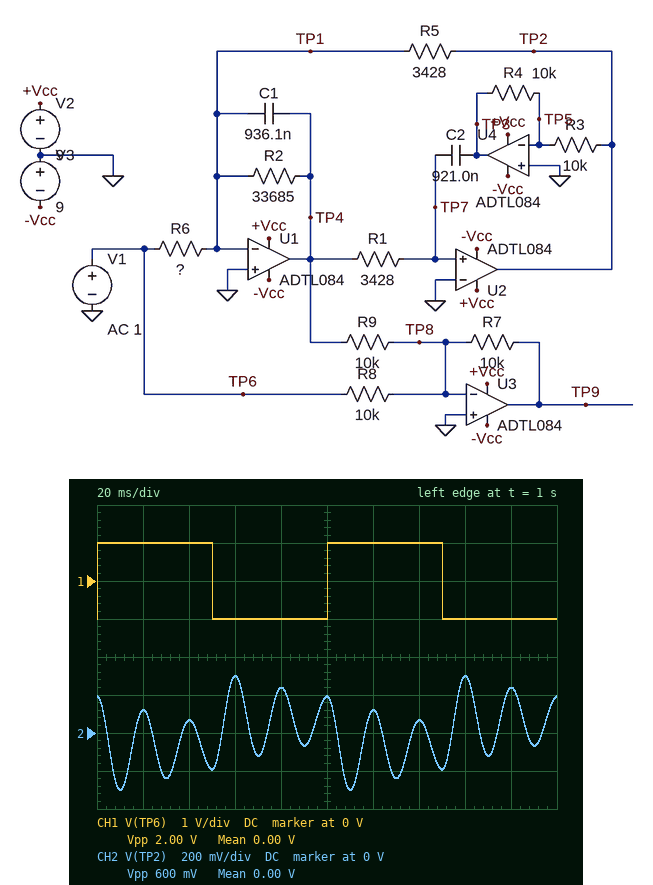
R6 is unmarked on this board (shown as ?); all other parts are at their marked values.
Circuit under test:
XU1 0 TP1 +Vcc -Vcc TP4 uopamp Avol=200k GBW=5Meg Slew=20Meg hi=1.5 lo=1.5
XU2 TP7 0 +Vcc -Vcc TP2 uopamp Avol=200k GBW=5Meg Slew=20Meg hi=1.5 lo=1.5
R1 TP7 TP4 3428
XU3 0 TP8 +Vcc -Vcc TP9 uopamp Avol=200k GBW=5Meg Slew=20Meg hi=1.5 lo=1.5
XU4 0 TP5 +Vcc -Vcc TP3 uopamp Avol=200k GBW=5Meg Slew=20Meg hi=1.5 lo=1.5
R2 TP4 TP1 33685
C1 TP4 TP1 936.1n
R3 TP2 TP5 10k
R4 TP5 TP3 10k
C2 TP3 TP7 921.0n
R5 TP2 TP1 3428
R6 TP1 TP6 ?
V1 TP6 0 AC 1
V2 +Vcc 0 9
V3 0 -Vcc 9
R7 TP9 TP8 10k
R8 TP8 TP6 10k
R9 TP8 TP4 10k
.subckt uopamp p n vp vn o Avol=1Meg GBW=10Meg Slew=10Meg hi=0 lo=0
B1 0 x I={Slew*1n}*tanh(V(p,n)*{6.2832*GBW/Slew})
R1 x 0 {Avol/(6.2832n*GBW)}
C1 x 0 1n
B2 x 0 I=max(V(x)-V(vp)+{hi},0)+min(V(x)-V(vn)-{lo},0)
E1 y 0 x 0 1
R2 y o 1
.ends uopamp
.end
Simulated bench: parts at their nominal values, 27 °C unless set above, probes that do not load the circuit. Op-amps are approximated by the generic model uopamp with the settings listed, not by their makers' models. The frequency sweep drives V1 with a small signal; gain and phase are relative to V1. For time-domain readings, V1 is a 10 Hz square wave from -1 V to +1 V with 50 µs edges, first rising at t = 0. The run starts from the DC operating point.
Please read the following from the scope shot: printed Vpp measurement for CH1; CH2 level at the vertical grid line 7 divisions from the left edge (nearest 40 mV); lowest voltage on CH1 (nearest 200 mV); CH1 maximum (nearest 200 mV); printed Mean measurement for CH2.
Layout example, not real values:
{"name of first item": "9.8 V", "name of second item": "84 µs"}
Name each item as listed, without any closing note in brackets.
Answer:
{"printed Vpp measurement for CH1": "2.00 V", "CH2 level at the vertical grid line 7 divisions from the left edge": "80 mV", "lowest voltage on CH1": "-1.0 V", "CH1 maximum": "1.0 V", "printed Mean measurement for CH2": "0.00 V"}
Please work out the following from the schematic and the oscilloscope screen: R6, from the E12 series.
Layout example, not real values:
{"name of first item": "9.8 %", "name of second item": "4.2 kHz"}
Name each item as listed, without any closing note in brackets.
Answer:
{"R6, from the E12 series": "47 kΩ"}
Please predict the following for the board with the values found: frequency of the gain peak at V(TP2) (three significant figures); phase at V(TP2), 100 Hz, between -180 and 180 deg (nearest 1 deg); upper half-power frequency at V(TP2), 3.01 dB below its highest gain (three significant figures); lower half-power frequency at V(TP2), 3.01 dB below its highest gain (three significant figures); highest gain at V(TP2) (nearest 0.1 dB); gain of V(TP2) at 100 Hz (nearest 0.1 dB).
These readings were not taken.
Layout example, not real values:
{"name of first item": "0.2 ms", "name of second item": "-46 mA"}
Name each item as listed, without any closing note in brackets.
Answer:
{"frequency of the gain peak at V(TP2)": "49.9 Hz", "phase at V(TP2), 100 Hz, between -180 and 180 deg": "4 deg", "upper half-power frequency at V(TP2), 3.01 dB below its highest gain": "52.3 Hz", "lower half-power frequency at V(TP2), 3.01 dB below its highest gain": "47.3 Hz", "highest gain at V(TP2)": "-2.8 dB", "gain of V(TP2) at 100 Hz": "-32.3 dB"}
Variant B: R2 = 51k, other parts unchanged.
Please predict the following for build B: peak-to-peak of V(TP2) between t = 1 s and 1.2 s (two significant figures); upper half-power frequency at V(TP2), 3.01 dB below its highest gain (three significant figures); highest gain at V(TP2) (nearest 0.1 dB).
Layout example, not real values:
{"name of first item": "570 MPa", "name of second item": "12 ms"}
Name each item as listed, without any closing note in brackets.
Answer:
{"peak-to-peak of V(TP2) between t = 1 s and 1.2 s": "790 mV", "upper half-power frequency at V(TP2), 3.01 dB below its highest gain": "51.6 Hz", "highest gain at V(TP2)": "0.8 dB"}
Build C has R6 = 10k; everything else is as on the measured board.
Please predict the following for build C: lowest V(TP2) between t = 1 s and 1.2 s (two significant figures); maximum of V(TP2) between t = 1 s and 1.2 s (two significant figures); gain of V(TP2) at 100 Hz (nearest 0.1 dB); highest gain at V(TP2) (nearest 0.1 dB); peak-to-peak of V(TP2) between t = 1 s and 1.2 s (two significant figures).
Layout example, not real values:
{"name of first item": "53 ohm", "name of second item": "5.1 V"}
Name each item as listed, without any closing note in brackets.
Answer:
{"lowest V(TP2) between t = 1 s and 1.2 s": "-1.4 V", "maximum of V(TP2) between t = 1 s and 1.2 s": "1.4 V", "gain of V(TP2) at 100 Hz": "-18.9 dB", "highest gain at V(TP2)": "10.6 dB", "peak-to-peak of V(TP2) between t = 1 s and 1.2 s": "2.8 V"}
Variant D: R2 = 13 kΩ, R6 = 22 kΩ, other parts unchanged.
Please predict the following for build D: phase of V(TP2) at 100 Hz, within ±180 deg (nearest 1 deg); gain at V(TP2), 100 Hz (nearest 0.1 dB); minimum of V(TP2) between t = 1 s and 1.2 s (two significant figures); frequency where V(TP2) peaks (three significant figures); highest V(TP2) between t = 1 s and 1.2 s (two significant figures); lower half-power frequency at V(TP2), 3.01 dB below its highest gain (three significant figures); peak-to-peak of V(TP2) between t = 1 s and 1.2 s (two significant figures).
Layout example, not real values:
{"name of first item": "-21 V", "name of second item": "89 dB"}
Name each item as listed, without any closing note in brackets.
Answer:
{"phase of V(TP2) at 100 Hz, within ±180 deg": "10 deg", "gain at V(TP2), 100 Hz": "-25.8 dB", "minimum of V(TP2) between t = 1 s and 1.2 s": "-390 mV", "frequency where V(TP2) peaks": "49.1 Hz", "highest V(TP2) between t = 1 s and 1.2 s": "390 mV", "lower half-power frequency at V(TP2), 3.01 dB below its highest gain": "42.0 Hz", "peak-to-peak of V(TP2) between t = 1 s and 1.2 s": "780 mV"}
